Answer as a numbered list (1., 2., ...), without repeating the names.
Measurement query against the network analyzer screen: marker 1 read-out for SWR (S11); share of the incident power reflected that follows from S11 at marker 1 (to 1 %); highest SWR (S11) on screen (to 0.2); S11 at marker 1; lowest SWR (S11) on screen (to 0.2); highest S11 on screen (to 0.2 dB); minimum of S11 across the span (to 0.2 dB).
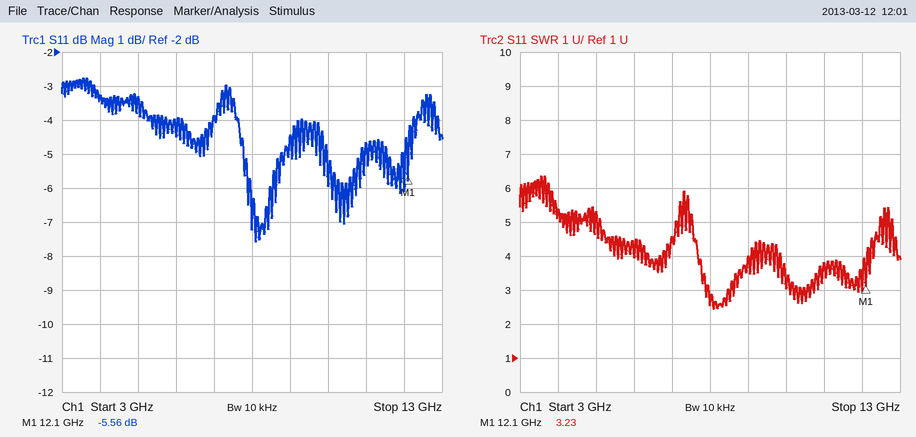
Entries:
1. 3.23
2. 28 %
3. 6.4
4. -5.56 dB
5. 2.4
6. -2.8 dB
7. -7.6 dB
